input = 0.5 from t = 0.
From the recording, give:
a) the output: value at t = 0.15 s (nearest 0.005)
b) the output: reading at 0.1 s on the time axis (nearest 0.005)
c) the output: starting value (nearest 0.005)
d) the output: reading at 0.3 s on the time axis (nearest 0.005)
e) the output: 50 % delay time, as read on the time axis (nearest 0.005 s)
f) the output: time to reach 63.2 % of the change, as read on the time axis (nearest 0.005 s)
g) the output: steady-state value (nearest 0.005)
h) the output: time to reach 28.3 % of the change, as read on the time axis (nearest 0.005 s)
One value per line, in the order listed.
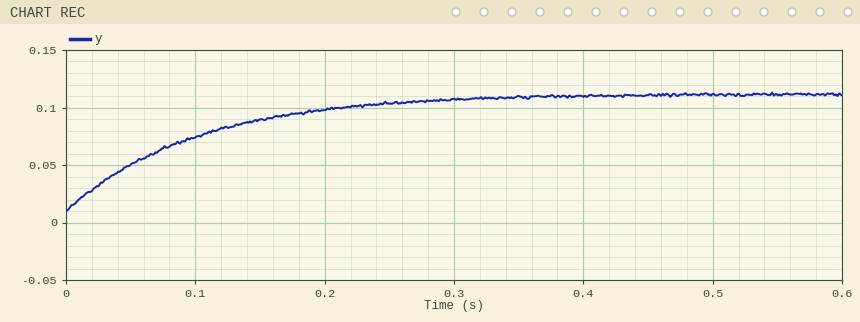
0.090
0.075
0.010
0.105
0.070 s
0.100 s
0.110
0.035 s
